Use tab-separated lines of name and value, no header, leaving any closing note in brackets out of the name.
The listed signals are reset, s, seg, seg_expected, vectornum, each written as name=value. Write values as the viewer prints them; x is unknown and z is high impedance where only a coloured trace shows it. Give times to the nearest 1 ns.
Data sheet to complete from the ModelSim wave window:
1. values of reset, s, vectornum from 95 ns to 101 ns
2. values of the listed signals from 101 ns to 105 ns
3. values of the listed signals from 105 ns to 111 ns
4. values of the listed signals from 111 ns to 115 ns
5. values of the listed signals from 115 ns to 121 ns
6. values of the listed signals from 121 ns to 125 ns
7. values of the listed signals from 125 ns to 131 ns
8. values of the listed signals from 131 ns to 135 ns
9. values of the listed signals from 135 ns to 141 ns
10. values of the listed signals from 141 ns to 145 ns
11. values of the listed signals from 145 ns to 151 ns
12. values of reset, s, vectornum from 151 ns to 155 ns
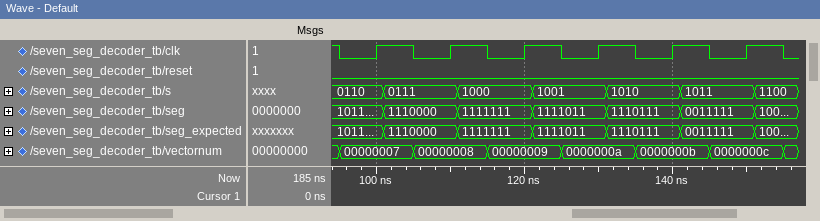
values of reset, s, vectornum from 95 ns to 101 ns	reset=0, s=0110, vectornum=00000007
values of the listed signals from 101 ns to 105 ns	reset=0, s=0111, seg=1110000, seg_expected=1110000, vectornum=00000007
values of the listed signals from 105 ns to 111 ns	reset=0, s=0111, seg=1110000, seg_expected=1110000, vectornum=00000008
values of the listed signals from 111 ns to 115 ns	reset=0, s=1000, seg=1111111, seg_expected=1111111, vectornum=00000008
values of the listed signals from 115 ns to 121 ns	reset=0, s=1000, seg=1111111, seg_expected=1111111, vectornum=00000009
values of the listed signals from 121 ns to 125 ns	reset=0, s=1001, seg=1111011, seg_expected=1111011, vectornum=00000009
values of the listed signals from 125 ns to 131 ns	reset=0, s=1001, seg=1111011, seg_expected=1111011, vectornum=0000000a
values of the listed signals from 131 ns to 135 ns	reset=0, s=1010, seg=1110111, seg_expected=1110111, vectornum=0000000a
values of the listed signals from 135 ns to 141 ns	reset=0, s=1010, seg=1110111, seg_expected=1110111, vectornum=0000000b
values of the listed signals from 141 ns to 145 ns	reset=0, s=1011, seg=0011111, seg_expected=0011111, vectornum=0000000b
values of the listed signals from 145 ns to 151 ns	reset=0, s=1011, seg=0011111, seg_expected=0011111, vectornum=0000000c
values of reset, s, vectornum from 151 ns to 155 ns	reset=0, s=1100, vectornum=0000000c
